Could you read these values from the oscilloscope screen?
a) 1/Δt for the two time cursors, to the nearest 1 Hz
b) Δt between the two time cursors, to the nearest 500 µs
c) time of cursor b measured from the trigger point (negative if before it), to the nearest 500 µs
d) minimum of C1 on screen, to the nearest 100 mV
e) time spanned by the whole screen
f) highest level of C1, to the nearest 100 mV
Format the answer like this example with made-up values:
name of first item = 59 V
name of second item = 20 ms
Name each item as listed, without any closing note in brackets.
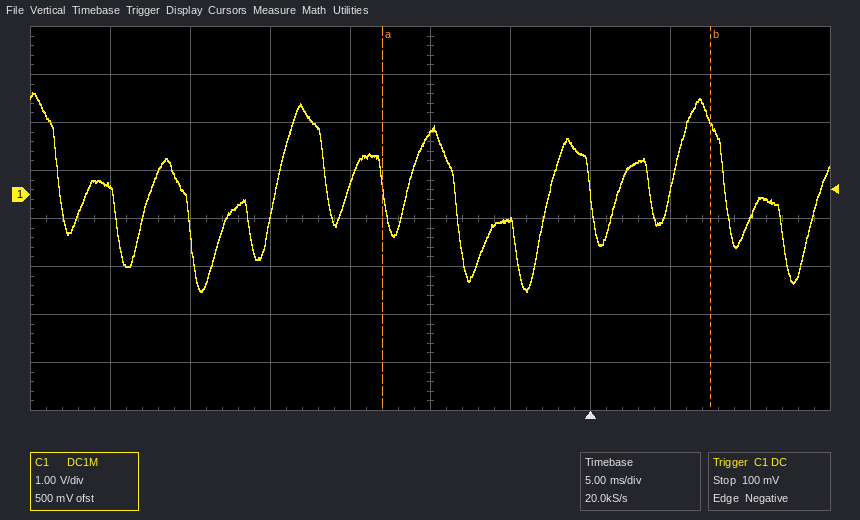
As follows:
1/Δt for the two time cursors, to the nearest 1 Hz = 49 Hz
Δt between the two time cursors, to the nearest 500 µs = 20.5 ms
time of cursor b measured from the trigger point (negative if before it), to the nearest 500 µs = +7.5 ms
minimum of C1 on screen, to the nearest 100 mV = -2.0 V
time spanned by the whole screen = 50 ms
highest level of C1, to the nearest 100 mV = 2.1 V
